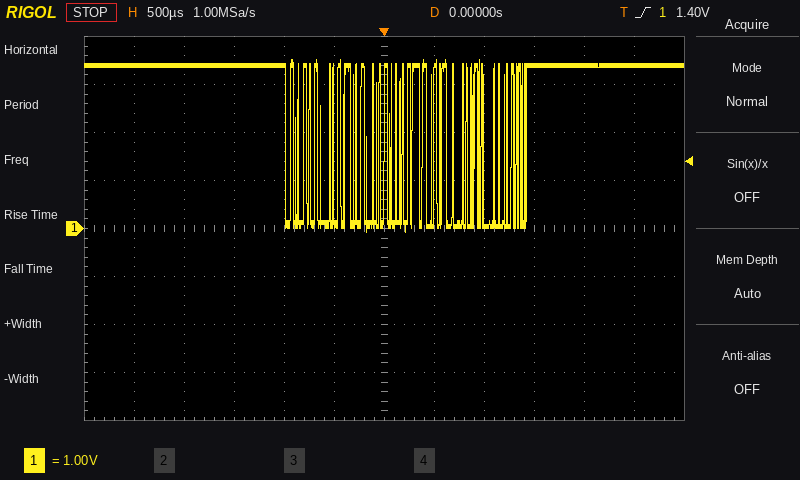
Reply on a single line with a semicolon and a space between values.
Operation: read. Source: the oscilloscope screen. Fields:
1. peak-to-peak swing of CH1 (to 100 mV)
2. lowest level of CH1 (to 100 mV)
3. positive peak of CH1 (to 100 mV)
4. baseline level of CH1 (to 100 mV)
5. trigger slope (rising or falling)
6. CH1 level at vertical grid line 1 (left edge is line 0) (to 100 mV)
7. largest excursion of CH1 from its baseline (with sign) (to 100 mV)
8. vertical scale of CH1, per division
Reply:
3.6 V; -100 mV; 3.5 V; 3.4 V; rising; 3.4 V; -3.5 V; 1 V
